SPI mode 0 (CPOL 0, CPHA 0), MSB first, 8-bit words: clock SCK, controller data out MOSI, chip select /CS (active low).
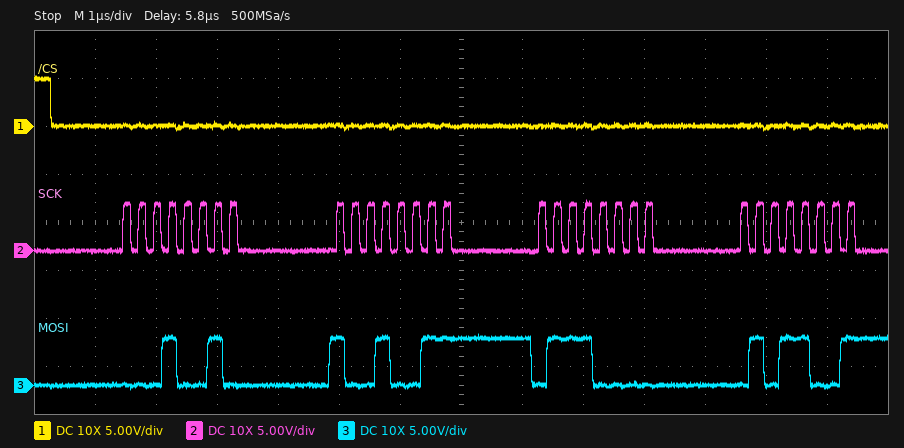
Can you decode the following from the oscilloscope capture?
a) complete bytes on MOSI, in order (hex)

12 93 70 59
